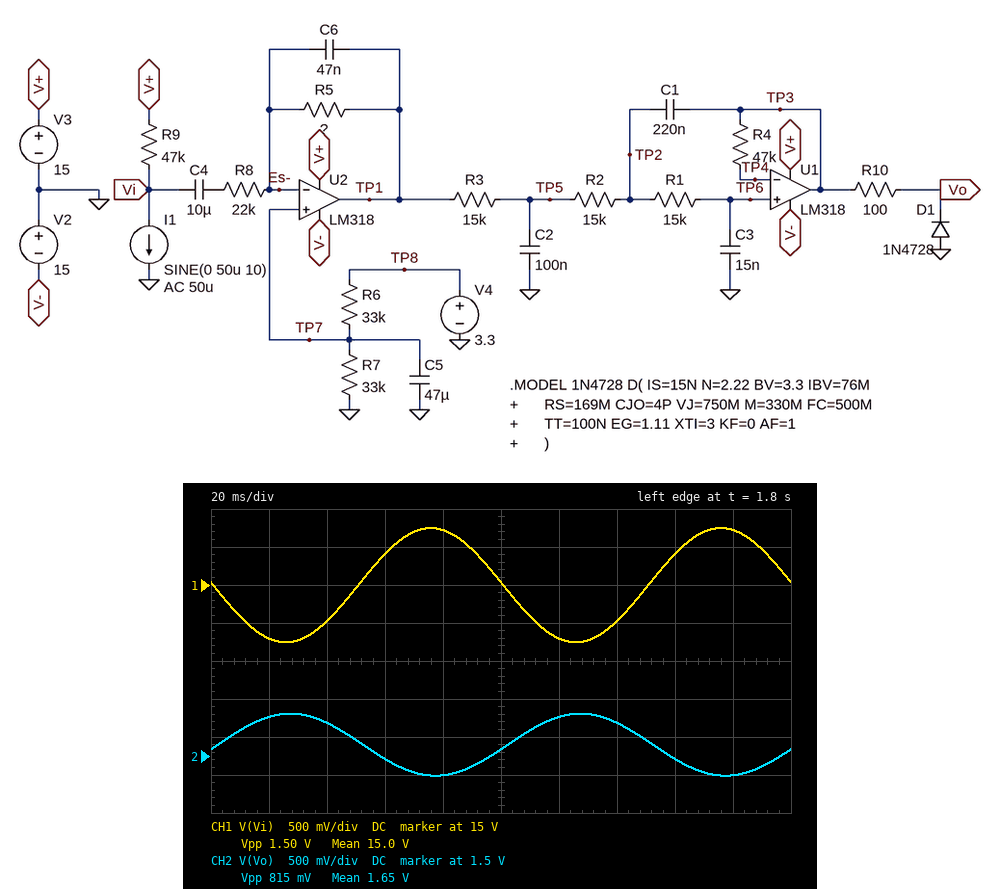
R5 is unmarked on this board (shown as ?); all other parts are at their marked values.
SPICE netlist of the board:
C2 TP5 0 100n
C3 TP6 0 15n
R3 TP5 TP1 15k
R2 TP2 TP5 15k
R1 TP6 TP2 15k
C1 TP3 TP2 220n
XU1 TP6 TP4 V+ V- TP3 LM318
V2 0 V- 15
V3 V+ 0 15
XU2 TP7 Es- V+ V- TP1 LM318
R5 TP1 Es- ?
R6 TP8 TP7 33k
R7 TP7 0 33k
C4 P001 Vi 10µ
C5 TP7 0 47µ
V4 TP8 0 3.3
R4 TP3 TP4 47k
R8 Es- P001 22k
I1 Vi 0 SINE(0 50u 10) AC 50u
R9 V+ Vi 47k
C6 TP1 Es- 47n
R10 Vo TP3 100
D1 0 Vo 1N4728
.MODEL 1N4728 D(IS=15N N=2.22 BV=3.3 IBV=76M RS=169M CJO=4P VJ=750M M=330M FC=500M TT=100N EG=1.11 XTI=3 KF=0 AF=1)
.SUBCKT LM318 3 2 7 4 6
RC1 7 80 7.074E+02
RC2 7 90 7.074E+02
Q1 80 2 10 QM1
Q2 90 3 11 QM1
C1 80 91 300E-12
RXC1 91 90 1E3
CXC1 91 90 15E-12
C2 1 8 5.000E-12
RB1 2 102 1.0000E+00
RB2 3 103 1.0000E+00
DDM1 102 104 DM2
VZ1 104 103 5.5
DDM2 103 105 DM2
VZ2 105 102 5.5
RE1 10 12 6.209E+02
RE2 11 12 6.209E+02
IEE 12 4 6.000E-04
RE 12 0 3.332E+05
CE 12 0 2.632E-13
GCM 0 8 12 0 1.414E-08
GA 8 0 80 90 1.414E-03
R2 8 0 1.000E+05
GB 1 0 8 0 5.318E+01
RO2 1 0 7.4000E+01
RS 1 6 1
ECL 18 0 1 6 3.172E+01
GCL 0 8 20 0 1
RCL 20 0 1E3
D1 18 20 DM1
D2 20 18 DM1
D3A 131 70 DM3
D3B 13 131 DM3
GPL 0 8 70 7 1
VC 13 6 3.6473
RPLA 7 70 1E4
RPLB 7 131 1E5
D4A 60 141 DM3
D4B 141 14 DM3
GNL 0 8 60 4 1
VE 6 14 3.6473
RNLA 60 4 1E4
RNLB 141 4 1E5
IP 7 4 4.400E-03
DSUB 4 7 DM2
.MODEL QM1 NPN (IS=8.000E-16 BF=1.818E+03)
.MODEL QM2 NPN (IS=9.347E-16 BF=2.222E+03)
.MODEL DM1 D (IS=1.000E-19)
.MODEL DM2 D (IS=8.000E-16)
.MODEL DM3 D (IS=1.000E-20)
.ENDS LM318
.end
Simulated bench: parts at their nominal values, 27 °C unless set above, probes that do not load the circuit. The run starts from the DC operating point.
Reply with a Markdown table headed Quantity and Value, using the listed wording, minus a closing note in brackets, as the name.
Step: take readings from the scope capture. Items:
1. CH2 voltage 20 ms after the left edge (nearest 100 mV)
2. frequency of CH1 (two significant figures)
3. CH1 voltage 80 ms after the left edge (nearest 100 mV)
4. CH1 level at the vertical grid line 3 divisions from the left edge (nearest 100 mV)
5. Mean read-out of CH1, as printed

| Quantity | Value |
|---|---|
| CH2 voltage 20 ms after the left edge | 2.0 V |
| frequency of CH1 | 10 Hz |
| CH1 voltage 80 ms after the left edge | 15.7 V |
| CH1 level at the vertical grid line 3 divisions from the left edge | 15.4 V |
| Mean read-out of CH1, as printed | 15.0 V |
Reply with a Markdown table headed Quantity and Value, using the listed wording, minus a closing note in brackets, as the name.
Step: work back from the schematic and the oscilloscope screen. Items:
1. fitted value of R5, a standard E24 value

| Quantity | Value |
|---|---|
| fitted value of R5, a standard E24 value | 12 kΩ |
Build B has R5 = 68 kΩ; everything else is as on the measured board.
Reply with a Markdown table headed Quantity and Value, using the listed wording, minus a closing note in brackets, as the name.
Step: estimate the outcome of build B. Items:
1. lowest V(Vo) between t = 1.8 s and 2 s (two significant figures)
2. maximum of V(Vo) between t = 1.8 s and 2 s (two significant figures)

| Quantity | Value |
|---|---|
| lowest V(Vo) between t = 1.8 s and 2 s | -580 mV |
| maximum of V(Vo) between t = 1.8 s and 2 s | 3.2 V |
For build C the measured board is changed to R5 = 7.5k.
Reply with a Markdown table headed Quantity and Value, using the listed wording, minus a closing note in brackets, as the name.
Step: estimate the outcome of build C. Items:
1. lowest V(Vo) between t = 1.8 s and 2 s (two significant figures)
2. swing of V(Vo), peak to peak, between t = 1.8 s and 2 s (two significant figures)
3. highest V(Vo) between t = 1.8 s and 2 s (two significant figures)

| Quantity | Value |
|---|---|
| lowest V(Vo) between t = 1.8 s and 2 s | 1.4 V |
| swing of V(Vo), peak to peak, between t = 1.8 s and 2 s | 510 mV |
| highest V(Vo) between t = 1.8 s and 2 s | 1.9 V |
